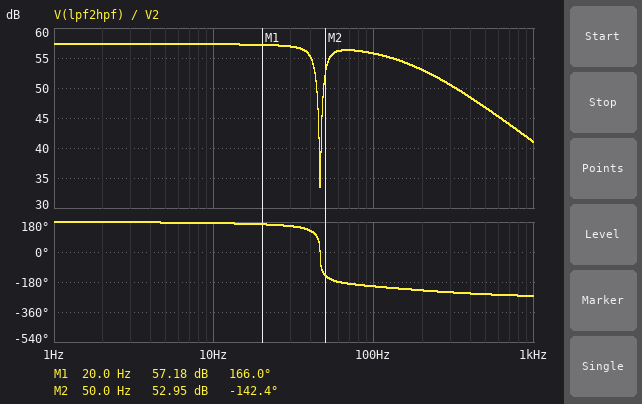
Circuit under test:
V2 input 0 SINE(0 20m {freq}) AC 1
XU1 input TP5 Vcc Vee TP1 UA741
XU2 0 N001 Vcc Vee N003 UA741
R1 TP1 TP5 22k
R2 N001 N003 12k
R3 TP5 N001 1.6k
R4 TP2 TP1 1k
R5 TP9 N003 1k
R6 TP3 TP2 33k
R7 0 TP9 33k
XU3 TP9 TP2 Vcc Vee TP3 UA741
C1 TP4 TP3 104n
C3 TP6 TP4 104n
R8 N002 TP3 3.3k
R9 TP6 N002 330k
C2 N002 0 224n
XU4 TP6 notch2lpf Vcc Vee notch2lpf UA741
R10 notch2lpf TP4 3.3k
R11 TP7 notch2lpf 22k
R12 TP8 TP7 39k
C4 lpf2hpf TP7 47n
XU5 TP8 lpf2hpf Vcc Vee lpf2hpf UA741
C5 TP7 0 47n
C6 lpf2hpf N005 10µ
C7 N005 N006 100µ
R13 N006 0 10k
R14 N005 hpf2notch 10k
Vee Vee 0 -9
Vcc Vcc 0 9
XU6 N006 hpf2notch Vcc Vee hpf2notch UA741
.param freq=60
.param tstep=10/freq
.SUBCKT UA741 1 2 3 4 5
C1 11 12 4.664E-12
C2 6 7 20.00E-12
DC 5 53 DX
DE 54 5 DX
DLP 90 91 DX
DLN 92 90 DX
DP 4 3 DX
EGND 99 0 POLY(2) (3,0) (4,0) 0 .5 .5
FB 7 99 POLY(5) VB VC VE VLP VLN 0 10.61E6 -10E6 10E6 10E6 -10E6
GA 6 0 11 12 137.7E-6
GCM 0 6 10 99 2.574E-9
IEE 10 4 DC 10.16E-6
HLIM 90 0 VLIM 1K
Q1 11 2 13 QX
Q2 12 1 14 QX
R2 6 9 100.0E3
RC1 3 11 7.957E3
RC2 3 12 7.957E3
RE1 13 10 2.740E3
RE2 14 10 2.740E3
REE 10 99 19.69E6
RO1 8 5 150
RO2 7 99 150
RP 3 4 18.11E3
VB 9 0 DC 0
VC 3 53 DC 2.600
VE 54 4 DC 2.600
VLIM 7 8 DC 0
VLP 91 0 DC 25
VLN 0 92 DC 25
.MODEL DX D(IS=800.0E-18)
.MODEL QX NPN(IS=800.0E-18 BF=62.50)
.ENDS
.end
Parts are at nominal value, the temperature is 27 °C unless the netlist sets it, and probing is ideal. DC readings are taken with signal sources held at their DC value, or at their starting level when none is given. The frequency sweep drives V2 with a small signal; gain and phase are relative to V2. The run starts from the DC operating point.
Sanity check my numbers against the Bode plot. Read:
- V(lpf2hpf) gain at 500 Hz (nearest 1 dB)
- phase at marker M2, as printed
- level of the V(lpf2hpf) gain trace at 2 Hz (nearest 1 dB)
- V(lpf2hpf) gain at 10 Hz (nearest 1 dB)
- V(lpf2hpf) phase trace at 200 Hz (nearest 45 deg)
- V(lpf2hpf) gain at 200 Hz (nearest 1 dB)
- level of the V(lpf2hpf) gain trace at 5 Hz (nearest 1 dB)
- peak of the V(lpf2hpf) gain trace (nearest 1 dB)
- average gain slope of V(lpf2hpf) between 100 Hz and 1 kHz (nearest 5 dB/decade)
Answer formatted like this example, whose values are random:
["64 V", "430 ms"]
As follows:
["47 dB", "-142.4 deg", "57 dB", "57 dB", "-225 deg", "53 dB", "57 dB", "57 dB", "-15 dB/decade"]
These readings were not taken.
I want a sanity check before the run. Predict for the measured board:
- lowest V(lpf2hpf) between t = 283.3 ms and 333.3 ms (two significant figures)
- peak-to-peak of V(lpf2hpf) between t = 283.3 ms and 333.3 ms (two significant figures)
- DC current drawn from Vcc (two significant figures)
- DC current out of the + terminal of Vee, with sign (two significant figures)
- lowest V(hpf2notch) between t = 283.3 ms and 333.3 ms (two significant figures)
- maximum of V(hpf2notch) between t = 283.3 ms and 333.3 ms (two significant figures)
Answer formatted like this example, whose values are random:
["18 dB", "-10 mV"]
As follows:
["-5.9 V", "12 V", "6.0 mA", "-6.0 mA", "-5.9 V", "6.0 V"]
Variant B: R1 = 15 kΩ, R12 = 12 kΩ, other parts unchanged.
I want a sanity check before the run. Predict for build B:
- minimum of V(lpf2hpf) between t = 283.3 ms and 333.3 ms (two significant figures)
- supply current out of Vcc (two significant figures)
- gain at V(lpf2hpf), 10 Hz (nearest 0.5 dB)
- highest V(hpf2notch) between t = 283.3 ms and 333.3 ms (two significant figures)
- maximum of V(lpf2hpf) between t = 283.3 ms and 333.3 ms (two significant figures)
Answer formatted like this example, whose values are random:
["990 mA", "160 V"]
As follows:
["-6.1 V", "6.0 mA", "55.5 dB", "6.2 V", "6.1 V"]
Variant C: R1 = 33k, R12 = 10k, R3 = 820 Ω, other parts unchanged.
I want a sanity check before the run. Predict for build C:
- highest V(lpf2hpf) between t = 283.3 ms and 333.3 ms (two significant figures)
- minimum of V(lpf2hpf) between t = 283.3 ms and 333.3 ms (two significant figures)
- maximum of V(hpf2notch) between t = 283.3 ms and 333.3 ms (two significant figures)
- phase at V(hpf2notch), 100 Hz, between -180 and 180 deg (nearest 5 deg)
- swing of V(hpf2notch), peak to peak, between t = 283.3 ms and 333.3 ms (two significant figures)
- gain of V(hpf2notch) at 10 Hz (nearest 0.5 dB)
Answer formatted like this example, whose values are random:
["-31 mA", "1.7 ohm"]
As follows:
["5.3 V", "-5.3 V", "5.4 V", "155 deg", "11 V", "65.0 dB"]
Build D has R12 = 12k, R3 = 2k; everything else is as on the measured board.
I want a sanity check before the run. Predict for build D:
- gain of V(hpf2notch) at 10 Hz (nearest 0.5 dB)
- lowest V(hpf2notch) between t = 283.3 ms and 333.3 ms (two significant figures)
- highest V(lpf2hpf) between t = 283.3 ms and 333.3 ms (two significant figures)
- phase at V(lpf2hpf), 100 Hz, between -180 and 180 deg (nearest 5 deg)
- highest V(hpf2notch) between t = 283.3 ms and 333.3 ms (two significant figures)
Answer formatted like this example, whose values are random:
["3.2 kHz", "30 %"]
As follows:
["55.5 dB", "-6.1 V", "6.1 V", "155 deg", "6.2 V"]
